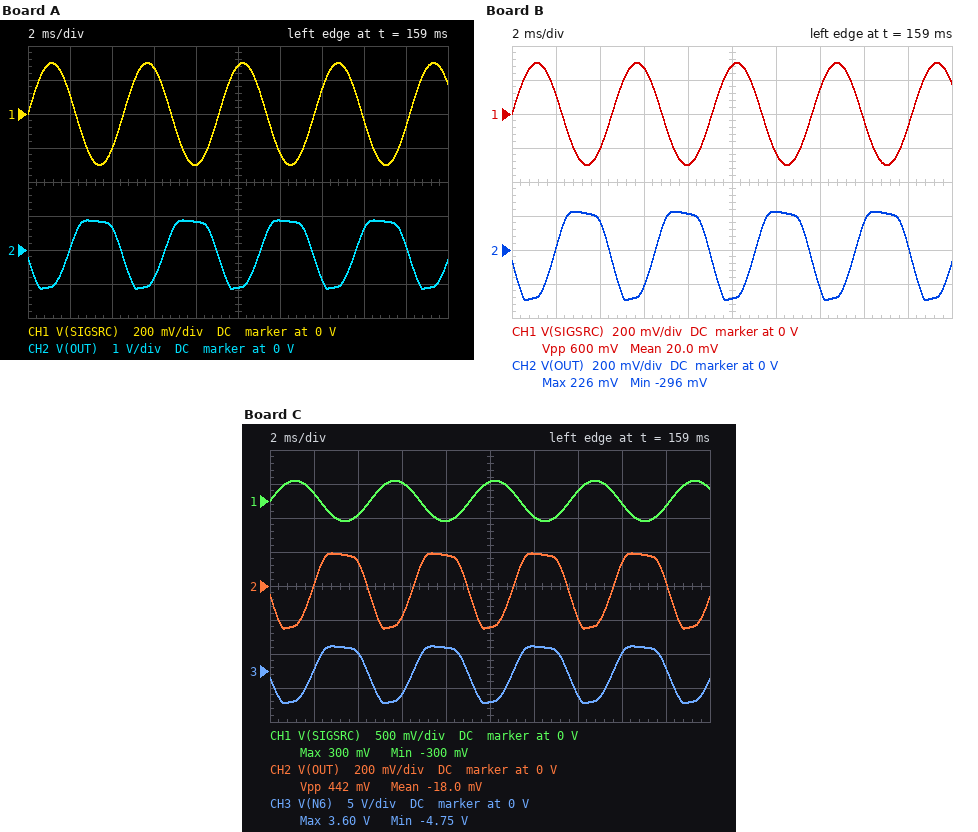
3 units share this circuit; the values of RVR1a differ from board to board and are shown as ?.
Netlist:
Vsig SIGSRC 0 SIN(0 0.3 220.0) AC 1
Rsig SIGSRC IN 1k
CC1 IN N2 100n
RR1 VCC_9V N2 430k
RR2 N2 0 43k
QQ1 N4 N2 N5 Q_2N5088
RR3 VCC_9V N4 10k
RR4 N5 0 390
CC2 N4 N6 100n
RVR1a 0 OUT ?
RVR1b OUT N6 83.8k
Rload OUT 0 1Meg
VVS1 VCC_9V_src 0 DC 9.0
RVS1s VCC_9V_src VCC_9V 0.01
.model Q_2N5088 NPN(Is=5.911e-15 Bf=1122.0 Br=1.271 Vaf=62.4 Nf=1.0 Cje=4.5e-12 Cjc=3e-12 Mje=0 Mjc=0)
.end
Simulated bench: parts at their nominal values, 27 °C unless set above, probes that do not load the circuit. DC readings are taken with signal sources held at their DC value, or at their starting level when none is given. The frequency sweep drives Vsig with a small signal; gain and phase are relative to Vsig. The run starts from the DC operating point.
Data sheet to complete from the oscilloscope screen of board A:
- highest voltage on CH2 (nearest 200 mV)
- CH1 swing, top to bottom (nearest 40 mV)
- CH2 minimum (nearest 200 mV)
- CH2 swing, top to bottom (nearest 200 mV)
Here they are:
800 mV
600 mV
-1.2 V
2.0 V
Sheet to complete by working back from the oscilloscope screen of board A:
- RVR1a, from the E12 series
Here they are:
27 kΩ
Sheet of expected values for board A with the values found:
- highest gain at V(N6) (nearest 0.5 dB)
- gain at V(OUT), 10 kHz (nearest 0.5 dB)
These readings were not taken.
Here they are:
26.0 dB
13.5 dB
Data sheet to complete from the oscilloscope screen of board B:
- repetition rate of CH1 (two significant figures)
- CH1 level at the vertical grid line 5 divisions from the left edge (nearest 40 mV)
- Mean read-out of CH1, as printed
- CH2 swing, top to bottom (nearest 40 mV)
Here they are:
220 Hz
280 mV
20.0 mV
520 mV
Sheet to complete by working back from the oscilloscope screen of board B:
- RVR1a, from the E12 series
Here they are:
5.6 kΩ
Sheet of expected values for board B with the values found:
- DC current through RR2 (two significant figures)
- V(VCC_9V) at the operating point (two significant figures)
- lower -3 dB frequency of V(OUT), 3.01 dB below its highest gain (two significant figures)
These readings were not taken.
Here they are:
19 µA
9.0 V
48 Hz
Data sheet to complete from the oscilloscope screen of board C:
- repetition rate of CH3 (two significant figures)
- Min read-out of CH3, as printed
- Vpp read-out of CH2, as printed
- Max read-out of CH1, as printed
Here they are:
220 Hz
-4.75 V
442 mV
300 mV
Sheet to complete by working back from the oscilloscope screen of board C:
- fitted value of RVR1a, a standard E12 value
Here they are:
4.7 kΩ
